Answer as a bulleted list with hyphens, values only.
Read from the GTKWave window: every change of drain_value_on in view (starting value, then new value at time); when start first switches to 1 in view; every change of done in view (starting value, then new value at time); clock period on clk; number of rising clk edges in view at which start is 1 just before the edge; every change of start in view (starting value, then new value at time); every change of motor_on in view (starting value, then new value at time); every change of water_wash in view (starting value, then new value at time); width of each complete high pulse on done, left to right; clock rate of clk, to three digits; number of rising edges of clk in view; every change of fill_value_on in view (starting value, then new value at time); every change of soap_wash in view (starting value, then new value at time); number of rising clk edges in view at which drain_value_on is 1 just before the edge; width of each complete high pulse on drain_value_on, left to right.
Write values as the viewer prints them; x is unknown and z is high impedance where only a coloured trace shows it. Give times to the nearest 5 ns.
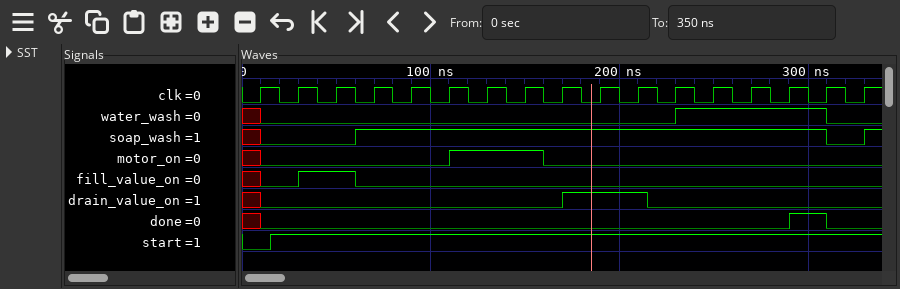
- x, 0 at 10 ns, 1 at 170 ns, 0 at 215 ns
- 15 ns
- x, 0 at 10 ns, 1 at 290 ns, 0 at 310 ns
- 20 ns
- 16
- 0, 1 at 15 ns
- x, 0 at 10 ns, 1 at 110 ns, 0 at 160 ns
- x, 0 at 10 ns, 1 at 230 ns, 0 at 310 ns
- 20 ns
- 50.0 MHz
- 17
- x, 0 at 10 ns, 1 at 30 ns, 0 at 60 ns
- x, 0 at 10 ns, 1 at 60 ns, 0 at 310 ns, 1 at 330 ns
- 2
- 45 ns
